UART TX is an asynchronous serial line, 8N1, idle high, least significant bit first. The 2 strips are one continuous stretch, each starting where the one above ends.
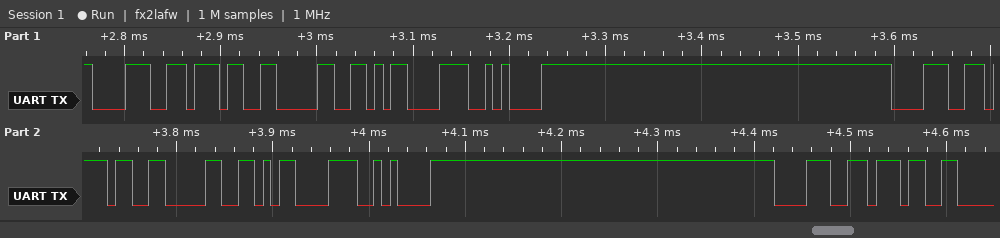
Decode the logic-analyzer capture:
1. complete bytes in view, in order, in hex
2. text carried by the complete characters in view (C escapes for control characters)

38 37 30 0D 0A 38 37 30 0D 0A 38 37
"870\r\n870\r\n87"
